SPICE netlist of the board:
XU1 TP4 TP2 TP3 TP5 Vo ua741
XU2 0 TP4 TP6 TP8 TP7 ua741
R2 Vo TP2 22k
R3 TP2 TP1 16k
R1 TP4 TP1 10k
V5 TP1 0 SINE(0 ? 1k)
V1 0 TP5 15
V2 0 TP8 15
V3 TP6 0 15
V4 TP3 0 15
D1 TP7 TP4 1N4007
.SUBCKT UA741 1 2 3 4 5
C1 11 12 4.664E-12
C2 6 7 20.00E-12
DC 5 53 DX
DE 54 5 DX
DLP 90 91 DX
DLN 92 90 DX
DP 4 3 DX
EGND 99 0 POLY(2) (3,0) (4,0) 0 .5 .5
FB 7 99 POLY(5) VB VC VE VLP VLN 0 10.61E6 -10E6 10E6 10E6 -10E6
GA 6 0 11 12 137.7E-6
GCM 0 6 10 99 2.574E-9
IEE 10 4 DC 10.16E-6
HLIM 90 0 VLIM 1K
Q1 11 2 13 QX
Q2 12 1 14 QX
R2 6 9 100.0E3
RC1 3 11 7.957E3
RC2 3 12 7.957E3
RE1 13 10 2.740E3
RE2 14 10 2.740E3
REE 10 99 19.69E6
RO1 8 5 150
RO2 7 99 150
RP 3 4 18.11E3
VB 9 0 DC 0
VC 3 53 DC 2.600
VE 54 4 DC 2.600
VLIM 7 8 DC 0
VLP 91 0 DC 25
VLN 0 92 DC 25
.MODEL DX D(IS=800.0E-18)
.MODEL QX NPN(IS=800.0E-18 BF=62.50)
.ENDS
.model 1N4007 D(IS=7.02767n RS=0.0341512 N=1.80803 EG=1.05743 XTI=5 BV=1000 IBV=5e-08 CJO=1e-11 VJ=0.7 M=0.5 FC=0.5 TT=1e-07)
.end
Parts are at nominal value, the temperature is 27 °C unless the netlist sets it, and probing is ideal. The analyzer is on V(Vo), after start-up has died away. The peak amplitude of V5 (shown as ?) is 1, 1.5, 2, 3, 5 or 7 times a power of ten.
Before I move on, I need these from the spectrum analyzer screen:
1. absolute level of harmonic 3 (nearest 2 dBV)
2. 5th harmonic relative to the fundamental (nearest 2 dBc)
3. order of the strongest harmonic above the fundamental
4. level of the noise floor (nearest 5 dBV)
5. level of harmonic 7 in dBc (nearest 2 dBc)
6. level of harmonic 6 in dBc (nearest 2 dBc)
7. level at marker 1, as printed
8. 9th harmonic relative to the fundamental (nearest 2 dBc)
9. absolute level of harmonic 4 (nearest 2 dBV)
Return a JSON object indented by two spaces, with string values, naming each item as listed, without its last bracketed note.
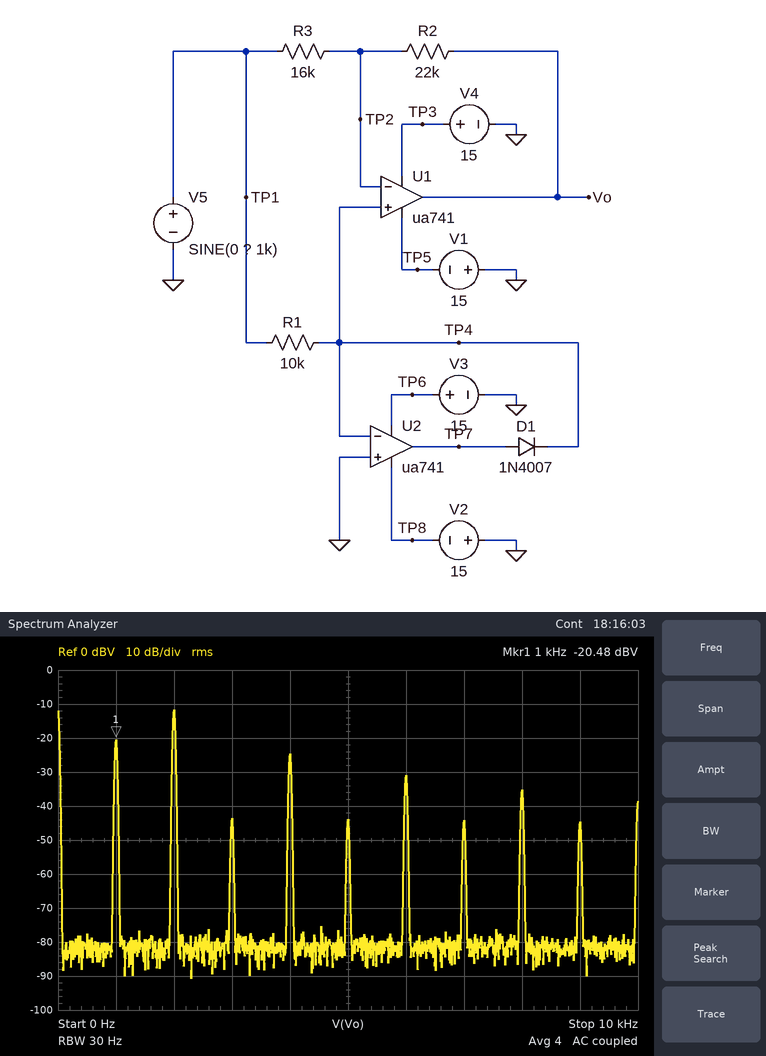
{
  "absolute level of harmonic 3": "-44 dBV",
  "5th harmonic relative to the fundamental": "-24 dBc",
  "order of the strongest harmonic above the fundamental": "2",
  "level of the noise floor": "-80 dBV",
  "level of harmonic 7 in dBc": "-24 dBc",
  "level of harmonic 6 in dBc": "-10 dBc",
  "level at marker 1, as printed": "-20.48 dBV",
  "9th harmonic relative to the fundamental": "-24 dBc",
  "absolute level of harmonic 4": "-24 dBV"
}
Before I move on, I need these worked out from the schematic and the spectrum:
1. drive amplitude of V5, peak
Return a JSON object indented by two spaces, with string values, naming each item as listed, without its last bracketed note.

{
  "drive amplitude of V5, peak": "700 mV"
}
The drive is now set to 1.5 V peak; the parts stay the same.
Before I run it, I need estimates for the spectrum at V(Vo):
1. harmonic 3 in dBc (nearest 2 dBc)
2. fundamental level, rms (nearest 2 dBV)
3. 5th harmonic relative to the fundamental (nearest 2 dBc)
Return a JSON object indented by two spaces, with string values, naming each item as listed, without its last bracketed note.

{
  "harmonic 3 in dBc": "-26 dBc",
  "fundamental level, rms": "-14 dBV",
  "5th harmonic relative to the fundamental": "-26 dBc"
}
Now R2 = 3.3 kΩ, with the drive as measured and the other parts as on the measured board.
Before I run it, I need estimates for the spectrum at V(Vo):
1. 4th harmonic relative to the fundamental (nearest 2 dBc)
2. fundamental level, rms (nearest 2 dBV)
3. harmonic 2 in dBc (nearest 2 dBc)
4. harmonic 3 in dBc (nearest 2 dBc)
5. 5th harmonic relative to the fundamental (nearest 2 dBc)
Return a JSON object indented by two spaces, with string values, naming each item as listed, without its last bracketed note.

{
  "4th harmonic relative to the fundamental": "-16 dBc",
  "fundamental level, rms": "-14 dBV",
  "harmonic 2 in dBc": "-4 dBc",
  "harmonic 3 in dBc": "-36 dBc",
  "5th harmonic relative to the fundamental": "-36 dBc"
}
